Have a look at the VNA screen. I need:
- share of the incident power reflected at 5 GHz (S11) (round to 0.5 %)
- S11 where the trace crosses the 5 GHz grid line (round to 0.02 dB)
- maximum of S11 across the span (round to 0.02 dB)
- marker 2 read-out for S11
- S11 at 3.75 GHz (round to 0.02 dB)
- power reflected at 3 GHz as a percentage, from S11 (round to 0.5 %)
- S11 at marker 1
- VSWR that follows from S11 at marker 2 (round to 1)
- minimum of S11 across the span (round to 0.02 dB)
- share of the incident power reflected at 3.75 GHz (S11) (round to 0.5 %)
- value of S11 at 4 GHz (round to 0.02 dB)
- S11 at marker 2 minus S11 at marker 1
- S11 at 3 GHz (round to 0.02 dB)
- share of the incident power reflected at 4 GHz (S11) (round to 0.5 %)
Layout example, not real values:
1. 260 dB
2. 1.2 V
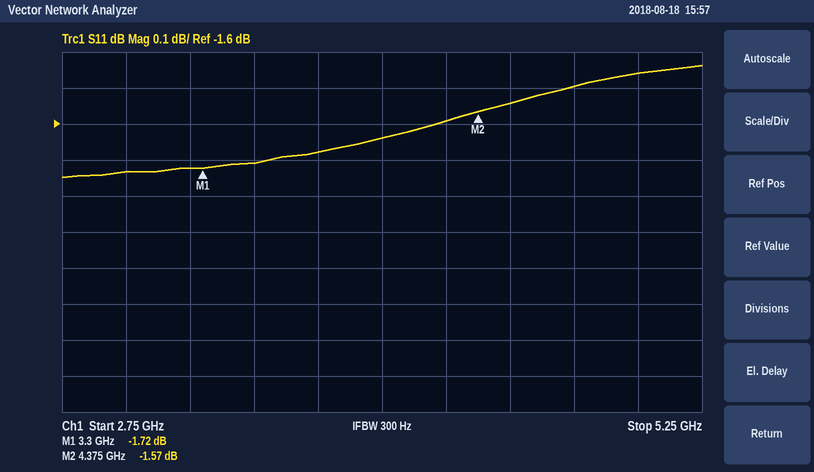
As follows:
1. 71.5 %
2. -1.46 dB
3. -1.44 dB
4. -1.57 dB
5. -1.68 dB
6. 67.0 %
7. -1.72 dB
8. 11
9. -1.74 dB
10. 68.0 %
11. -1.64 dB
12. 0.15 dB
13. -1.74 dB
14. 68.5 %
